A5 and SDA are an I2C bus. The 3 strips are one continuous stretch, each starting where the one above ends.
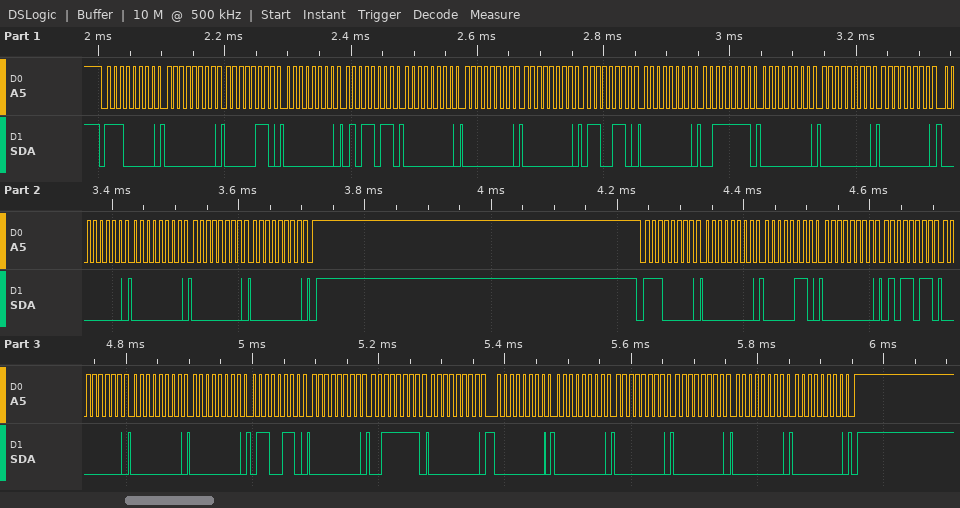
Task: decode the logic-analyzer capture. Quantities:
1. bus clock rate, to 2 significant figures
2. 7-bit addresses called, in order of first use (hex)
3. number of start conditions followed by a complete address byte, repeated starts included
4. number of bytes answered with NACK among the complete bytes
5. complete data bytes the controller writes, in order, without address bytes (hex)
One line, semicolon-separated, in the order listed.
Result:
100 kHz; 0x70; 2; 0; 00 06 00 5B 00 00 00 66 00 3F 00 00 00 00 00 00 00 00 06 00 5B 00 00 00 66 00 3F 00 00 00 00 00 00 00
